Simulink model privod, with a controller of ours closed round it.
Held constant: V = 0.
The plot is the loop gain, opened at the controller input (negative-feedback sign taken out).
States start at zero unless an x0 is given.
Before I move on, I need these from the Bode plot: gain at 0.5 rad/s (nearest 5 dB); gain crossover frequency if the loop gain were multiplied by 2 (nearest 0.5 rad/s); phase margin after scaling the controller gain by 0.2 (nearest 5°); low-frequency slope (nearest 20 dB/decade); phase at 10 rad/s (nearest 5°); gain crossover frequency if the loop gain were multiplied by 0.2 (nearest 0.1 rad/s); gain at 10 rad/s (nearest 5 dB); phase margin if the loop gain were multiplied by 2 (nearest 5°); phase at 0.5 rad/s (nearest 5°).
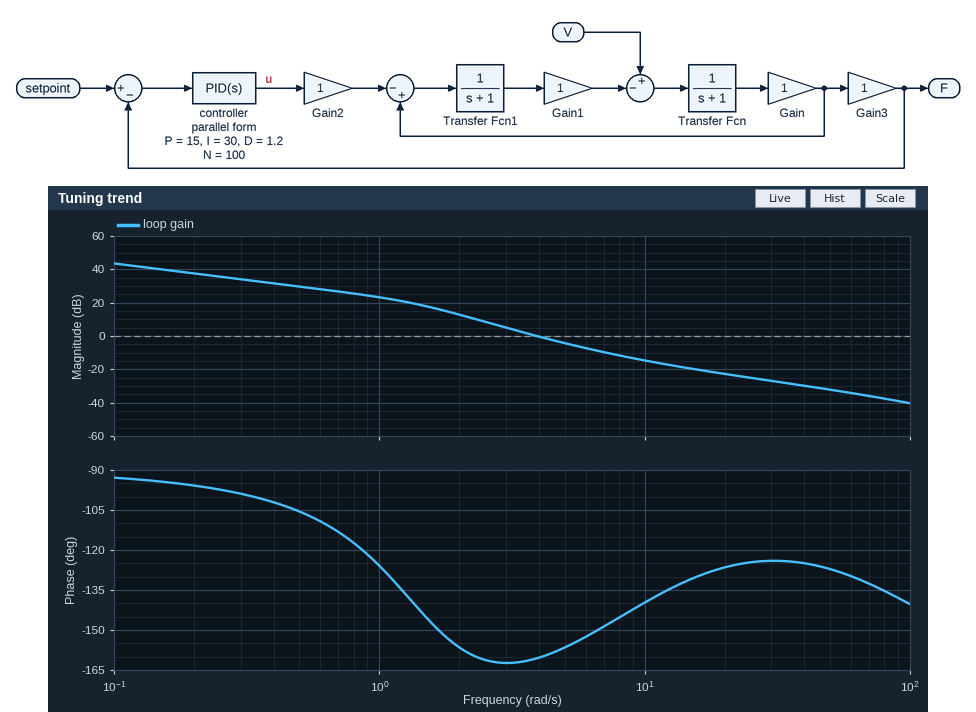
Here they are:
30 dB
5.5 rad/s
25°
-20 dB/decade
-140°
1.9 rad/s
-15 dB
25°
-105°
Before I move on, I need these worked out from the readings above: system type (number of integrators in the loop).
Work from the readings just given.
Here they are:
1
